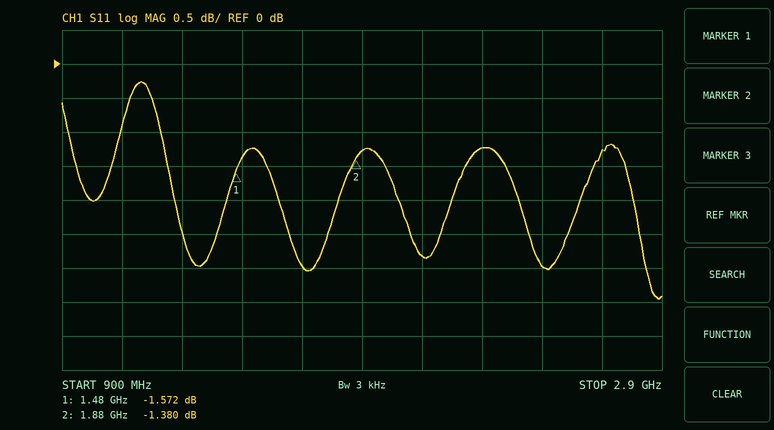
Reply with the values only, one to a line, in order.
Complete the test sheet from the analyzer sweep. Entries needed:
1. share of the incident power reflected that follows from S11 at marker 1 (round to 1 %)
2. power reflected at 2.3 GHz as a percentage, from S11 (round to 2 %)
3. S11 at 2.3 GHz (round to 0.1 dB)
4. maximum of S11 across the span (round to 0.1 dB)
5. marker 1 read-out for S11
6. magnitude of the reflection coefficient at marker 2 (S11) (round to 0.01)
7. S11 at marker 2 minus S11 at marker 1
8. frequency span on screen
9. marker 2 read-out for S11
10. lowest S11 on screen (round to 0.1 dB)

70 %
76 %
-1.2 dB
-0.3 dB
-1.572 dB
0.85
0.192 dB
2 GHz
-1.380 dB
-3.5 dB
